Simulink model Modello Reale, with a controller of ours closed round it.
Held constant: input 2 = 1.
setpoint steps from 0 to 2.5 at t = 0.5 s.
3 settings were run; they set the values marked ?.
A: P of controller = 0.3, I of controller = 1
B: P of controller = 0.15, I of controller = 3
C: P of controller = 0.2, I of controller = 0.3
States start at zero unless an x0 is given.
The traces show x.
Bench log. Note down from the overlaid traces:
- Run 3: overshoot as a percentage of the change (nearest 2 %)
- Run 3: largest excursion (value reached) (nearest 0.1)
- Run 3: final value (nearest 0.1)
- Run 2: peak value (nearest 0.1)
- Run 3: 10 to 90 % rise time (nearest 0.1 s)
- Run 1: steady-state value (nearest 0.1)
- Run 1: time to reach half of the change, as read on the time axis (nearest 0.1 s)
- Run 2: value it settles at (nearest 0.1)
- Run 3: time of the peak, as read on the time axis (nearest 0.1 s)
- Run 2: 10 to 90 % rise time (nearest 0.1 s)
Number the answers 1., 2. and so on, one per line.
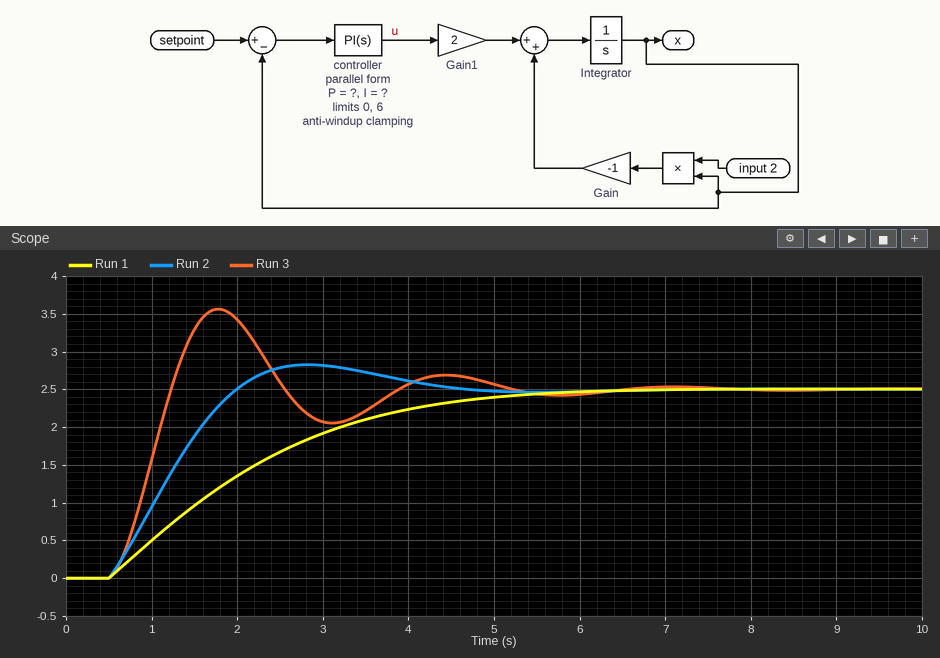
1. 42 %
2. 3.6
3. 2.5
4. 2.8
5. 0.5 s
6. 2.5
7. 1.9 s
8. 2.5
9. 1.8 s
10. 1.1 s
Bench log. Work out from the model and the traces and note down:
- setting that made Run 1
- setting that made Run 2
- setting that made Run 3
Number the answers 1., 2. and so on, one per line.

1. C
2. A
3. B
